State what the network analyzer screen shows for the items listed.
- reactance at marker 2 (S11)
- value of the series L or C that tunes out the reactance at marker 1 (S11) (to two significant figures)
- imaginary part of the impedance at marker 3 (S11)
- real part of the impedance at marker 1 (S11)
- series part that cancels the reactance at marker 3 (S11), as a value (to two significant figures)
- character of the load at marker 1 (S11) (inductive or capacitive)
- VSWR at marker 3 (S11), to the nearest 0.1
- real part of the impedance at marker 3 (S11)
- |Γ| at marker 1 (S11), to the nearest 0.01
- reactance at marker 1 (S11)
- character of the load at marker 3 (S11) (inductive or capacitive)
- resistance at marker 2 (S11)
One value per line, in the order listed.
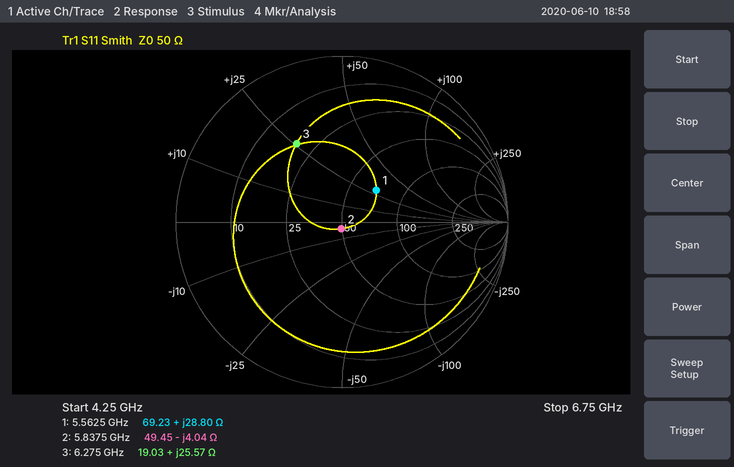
-4.04 Ω
990 fF
+25.57 Ω
69.23 Ω
990 fF
inductive
3.4
19.03 Ω
0.28
+28.80 Ω
inductive
49.45 Ω
